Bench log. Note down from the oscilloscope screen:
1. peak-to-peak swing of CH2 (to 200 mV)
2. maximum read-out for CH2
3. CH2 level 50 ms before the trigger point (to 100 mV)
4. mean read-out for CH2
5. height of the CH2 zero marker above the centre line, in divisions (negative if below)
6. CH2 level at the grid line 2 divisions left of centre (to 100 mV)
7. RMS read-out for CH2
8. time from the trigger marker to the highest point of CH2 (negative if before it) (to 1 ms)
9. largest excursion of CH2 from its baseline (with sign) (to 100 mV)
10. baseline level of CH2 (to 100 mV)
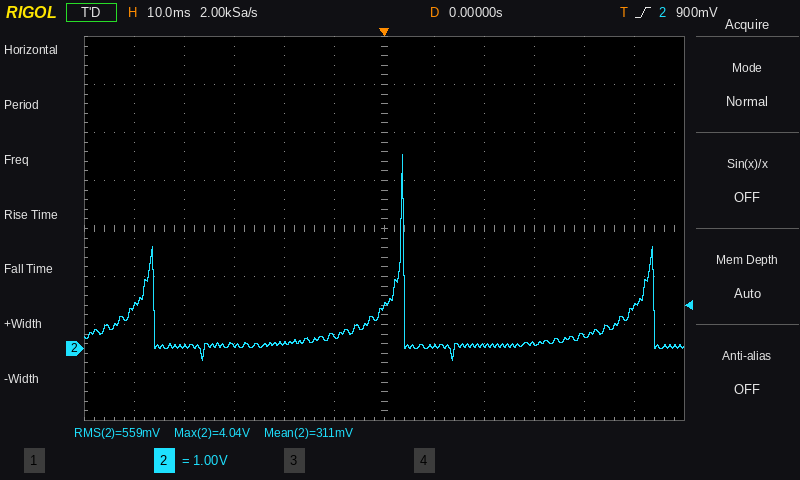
4.2 V
4.04 V
900 mV
311 mV
-2.5 div
100 mV
559 mV
+4 ms
+4.0 V
100 mV
